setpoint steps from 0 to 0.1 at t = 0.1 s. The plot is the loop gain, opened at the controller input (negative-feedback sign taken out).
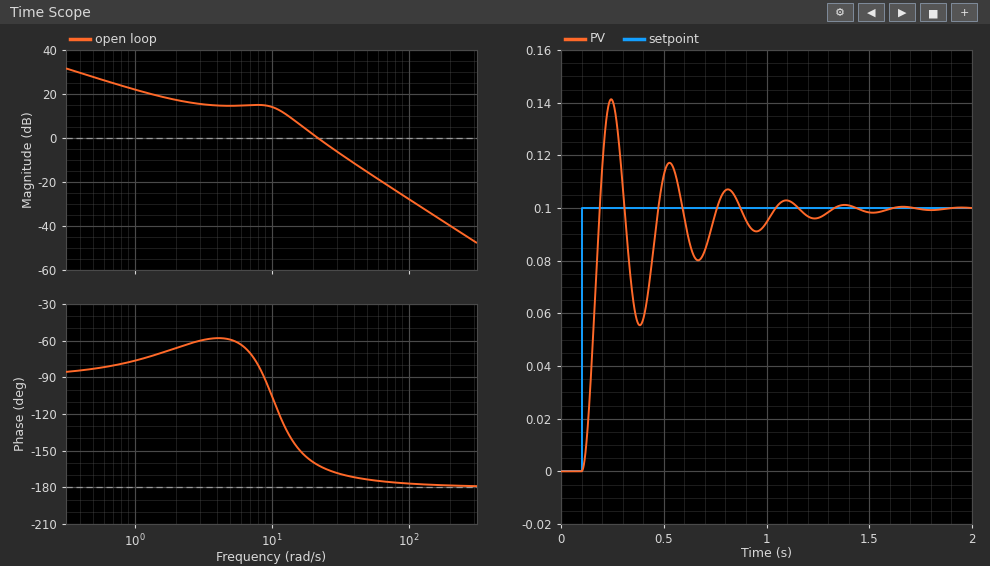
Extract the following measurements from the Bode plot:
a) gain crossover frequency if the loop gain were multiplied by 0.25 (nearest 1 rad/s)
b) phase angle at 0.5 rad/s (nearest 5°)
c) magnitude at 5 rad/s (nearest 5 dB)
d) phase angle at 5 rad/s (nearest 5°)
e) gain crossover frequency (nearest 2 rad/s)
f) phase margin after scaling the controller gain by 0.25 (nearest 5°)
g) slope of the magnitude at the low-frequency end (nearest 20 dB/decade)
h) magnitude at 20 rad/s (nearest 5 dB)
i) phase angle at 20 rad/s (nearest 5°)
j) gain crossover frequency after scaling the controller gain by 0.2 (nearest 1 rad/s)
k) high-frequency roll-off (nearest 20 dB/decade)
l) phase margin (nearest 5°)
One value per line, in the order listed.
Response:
12 rad/s
-85°
15 dB
-60°
22 rad/s
55°
-20 dB/decade
0 dB
-160°
10 rad/s
-40 dB/decade
20°
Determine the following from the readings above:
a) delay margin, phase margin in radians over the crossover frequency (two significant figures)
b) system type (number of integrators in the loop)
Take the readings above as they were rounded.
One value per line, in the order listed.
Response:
0.016 s
1
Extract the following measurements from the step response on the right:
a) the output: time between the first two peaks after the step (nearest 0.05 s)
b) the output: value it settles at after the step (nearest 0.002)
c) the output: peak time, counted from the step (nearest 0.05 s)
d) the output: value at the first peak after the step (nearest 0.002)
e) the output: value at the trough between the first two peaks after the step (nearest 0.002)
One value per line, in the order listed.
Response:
0.30 s
0.100
0.15 s
0.142
0.056
